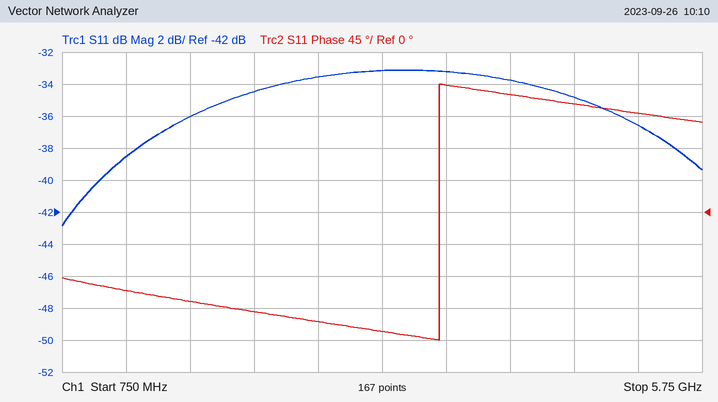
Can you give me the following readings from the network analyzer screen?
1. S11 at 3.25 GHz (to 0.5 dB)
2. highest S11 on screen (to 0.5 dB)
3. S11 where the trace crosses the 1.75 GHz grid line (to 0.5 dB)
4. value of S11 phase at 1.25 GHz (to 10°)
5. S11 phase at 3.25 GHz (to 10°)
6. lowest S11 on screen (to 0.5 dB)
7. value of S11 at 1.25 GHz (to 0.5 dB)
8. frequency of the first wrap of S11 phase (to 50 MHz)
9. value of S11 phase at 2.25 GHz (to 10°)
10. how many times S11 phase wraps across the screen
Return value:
-33.0 dB
-33.0 dB
-36.0 dB
-110°
-170°
-43.0 dB
-38.5 dB
3.70 GHz
-140°
1
